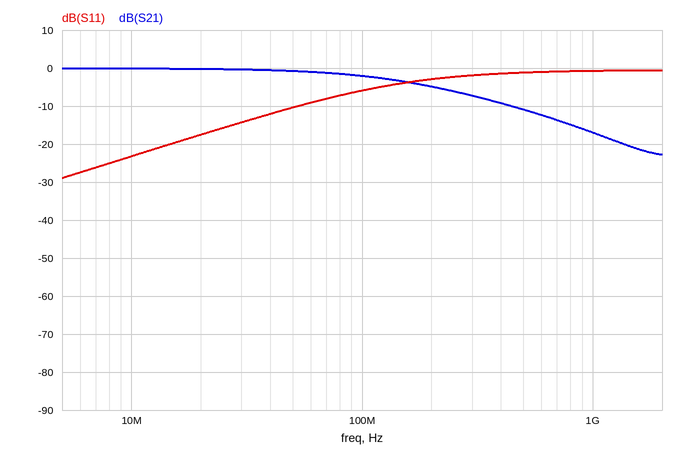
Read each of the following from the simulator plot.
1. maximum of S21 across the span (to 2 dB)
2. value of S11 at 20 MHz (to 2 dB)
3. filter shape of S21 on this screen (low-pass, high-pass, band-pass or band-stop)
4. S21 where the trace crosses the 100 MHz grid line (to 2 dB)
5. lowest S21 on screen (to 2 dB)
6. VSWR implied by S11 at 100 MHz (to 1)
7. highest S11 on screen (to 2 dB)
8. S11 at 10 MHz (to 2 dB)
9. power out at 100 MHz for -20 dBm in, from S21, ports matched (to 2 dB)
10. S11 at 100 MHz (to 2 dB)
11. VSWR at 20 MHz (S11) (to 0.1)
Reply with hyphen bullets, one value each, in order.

- 0 dB
- -18 dB
- low-pass
- -2 dB
- -22 dB
- 3
- 0 dB
- -24 dB
- -22 dBm
- -6 dB
- 1.3
